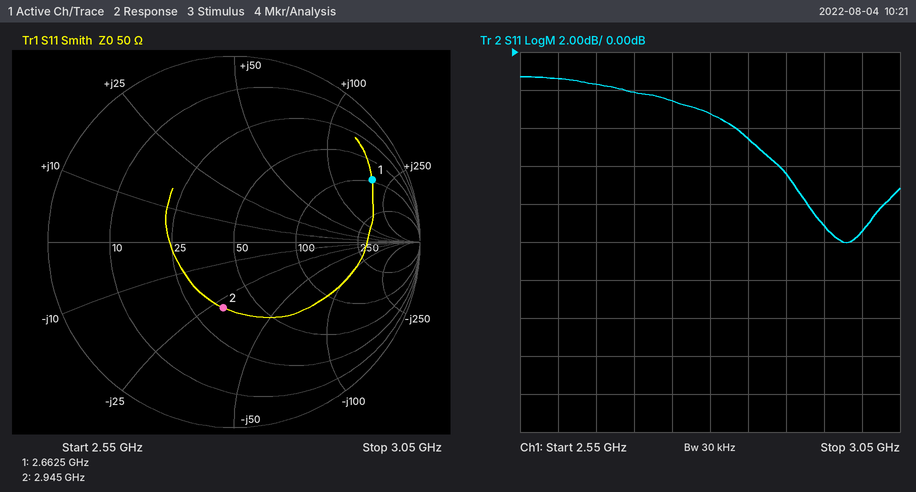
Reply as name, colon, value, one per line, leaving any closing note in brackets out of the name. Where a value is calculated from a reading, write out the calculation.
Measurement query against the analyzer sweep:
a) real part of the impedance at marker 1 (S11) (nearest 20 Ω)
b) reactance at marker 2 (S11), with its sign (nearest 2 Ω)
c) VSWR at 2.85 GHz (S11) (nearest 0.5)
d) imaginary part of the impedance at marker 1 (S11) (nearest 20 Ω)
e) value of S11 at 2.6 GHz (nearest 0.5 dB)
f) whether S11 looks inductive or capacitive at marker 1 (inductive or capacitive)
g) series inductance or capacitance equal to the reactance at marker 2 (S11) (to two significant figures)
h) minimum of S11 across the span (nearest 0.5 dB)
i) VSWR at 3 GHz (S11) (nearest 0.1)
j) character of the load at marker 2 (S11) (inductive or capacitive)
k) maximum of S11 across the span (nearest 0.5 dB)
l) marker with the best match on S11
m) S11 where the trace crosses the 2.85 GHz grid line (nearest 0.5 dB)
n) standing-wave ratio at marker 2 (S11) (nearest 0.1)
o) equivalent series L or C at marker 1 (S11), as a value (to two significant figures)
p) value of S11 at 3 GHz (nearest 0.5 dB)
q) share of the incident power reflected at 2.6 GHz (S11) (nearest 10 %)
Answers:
real part of the impedance at marker 1 (S11): 100 Ω
reactance at marker 2 (S11), with its sign: -28 Ω
VSWR at 2.85 GHz (S11): |Γ| = 10^(-4.5/20) = 0.5957; VSWR = (1 + 0.5957)/(1 − 0.5957) ≈ 4.0
imaginary part of the impedance at marker 1 (S11): +180 Ω
value of S11 at 2.6 GHz: -1.5 dB
whether S11 looks inductive or capacitive at marker 1: inductive
series inductance or capacitance equal to the reactance at marker 2 (S11): C = 1/(2π × 2.945 GHz × 28 Ω) ≈ 1.9 pF
minimum of S11 across the span: -10.0 dB
VSWR at 3 GHz (S11): |Γ| = 10^(-9.5/20) = 0.3350; VSWR = (1 + 0.3350)/(1 − 0.3350) ≈ 2.0
character of the load at marker 2 (S11): capacitive
maximum of S11 across the span: -1.5 dB
marker with the best match on S11: marker 2
S11 where the trace crosses the 2.85 GHz grid line: -4.5 dB
standing-wave ratio at marker 2 (S11): 2.1
equivalent series L or C at marker 1 (S11), as a value: L = 180 Ω/(2π × 2.6625 GHz) ≈ 11 nH
value of S11 at 3 GHz: -9.5 dB
share of the incident power reflected at 2.6 GHz (S11): 10^(-1.5/10) ≈ 70.8 %, so 70 % to the nearest 10 %
